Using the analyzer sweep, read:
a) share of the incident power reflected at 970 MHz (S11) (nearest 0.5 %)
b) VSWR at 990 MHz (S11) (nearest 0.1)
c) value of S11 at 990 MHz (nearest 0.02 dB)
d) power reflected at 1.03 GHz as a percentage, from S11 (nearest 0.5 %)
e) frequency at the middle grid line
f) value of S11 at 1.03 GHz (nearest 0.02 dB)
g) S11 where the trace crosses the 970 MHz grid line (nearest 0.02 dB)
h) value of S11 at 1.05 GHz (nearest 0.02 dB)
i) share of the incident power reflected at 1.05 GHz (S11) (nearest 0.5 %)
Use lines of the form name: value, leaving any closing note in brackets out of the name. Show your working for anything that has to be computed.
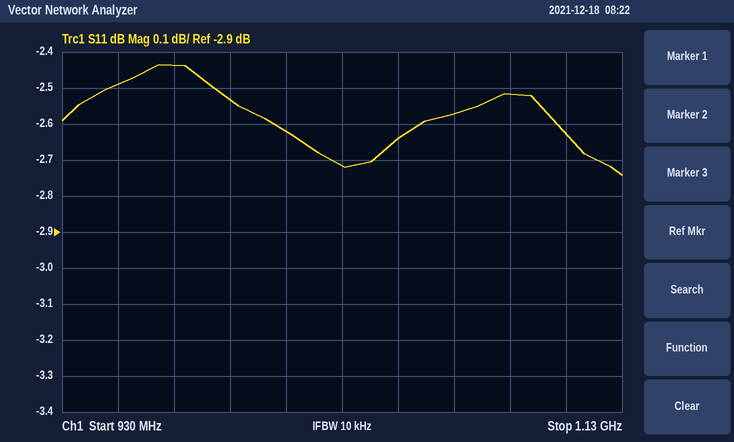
share of the incident power reflected at 970 MHz (S11): 10^(-2.44/10) ≈ 57.0 %
VSWR at 990 MHz (S11): |Γ| = 10^(-2.54/20) = 0.7464; VSWR = (1 + 0.7464)/(1 − 0.7464) ≈ 6.9
value of S11 at 990 MHz: -2.54 dB
power reflected at 1.03 GHz as a percentage, from S11: 10^(-2.72/10) ≈ 53.5 %
frequency at the middle grid line: 1.03 GHz
value of S11 at 1.03 GHz: -2.72 dB
S11 where the trace crosses the 970 MHz grid line: -2.44 dB
value of S11 at 1.05 GHz: -2.64 dB
share of the incident power reflected at 1.05 GHz (S11): 10^(-2.64/10) ≈ 54.5 %
